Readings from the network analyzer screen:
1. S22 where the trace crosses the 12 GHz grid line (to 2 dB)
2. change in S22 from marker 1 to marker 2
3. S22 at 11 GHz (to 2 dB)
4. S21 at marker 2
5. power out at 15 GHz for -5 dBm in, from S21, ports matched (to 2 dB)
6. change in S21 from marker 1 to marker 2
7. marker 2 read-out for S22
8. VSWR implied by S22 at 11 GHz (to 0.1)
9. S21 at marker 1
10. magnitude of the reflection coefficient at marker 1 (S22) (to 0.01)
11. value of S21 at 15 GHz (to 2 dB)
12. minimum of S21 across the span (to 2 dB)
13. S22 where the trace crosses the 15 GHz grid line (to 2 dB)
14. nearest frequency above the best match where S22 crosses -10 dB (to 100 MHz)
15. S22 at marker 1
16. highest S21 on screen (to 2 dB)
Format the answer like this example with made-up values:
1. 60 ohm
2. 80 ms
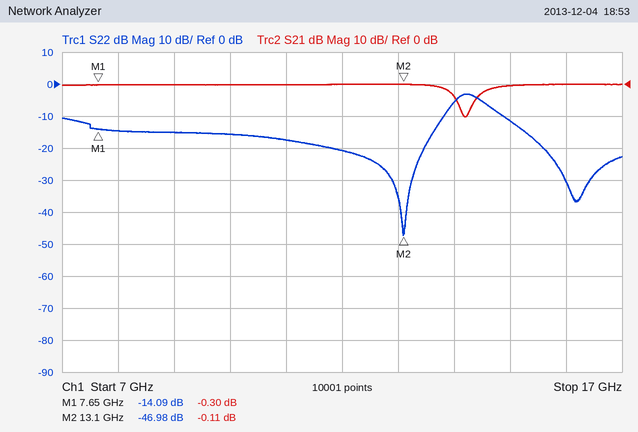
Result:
1. -20 dB
2. -32.89 dB
3. -18 dB
4. -0.11 dB
5. -6 dBm
6. 0.19 dB
7. -46.98 dB
8. 1.3
9. -0.30 dB
10. 0.20
11. 0 dB
12. -10 dB
13. -12 dB
14. 13.8 GHz
15. -14.09 dB
16. 0 dB
